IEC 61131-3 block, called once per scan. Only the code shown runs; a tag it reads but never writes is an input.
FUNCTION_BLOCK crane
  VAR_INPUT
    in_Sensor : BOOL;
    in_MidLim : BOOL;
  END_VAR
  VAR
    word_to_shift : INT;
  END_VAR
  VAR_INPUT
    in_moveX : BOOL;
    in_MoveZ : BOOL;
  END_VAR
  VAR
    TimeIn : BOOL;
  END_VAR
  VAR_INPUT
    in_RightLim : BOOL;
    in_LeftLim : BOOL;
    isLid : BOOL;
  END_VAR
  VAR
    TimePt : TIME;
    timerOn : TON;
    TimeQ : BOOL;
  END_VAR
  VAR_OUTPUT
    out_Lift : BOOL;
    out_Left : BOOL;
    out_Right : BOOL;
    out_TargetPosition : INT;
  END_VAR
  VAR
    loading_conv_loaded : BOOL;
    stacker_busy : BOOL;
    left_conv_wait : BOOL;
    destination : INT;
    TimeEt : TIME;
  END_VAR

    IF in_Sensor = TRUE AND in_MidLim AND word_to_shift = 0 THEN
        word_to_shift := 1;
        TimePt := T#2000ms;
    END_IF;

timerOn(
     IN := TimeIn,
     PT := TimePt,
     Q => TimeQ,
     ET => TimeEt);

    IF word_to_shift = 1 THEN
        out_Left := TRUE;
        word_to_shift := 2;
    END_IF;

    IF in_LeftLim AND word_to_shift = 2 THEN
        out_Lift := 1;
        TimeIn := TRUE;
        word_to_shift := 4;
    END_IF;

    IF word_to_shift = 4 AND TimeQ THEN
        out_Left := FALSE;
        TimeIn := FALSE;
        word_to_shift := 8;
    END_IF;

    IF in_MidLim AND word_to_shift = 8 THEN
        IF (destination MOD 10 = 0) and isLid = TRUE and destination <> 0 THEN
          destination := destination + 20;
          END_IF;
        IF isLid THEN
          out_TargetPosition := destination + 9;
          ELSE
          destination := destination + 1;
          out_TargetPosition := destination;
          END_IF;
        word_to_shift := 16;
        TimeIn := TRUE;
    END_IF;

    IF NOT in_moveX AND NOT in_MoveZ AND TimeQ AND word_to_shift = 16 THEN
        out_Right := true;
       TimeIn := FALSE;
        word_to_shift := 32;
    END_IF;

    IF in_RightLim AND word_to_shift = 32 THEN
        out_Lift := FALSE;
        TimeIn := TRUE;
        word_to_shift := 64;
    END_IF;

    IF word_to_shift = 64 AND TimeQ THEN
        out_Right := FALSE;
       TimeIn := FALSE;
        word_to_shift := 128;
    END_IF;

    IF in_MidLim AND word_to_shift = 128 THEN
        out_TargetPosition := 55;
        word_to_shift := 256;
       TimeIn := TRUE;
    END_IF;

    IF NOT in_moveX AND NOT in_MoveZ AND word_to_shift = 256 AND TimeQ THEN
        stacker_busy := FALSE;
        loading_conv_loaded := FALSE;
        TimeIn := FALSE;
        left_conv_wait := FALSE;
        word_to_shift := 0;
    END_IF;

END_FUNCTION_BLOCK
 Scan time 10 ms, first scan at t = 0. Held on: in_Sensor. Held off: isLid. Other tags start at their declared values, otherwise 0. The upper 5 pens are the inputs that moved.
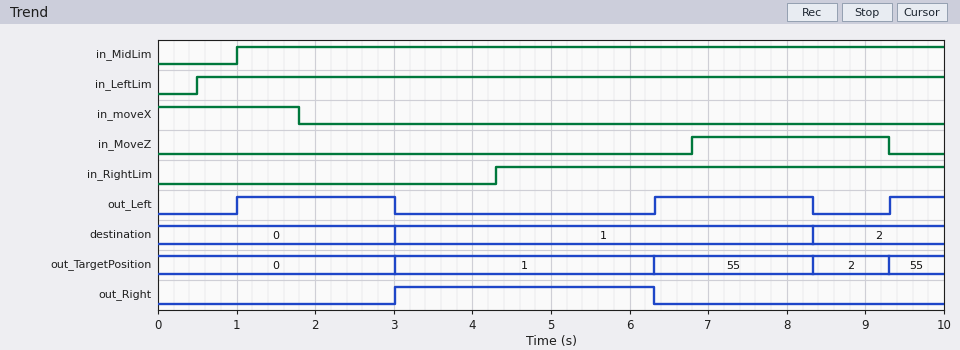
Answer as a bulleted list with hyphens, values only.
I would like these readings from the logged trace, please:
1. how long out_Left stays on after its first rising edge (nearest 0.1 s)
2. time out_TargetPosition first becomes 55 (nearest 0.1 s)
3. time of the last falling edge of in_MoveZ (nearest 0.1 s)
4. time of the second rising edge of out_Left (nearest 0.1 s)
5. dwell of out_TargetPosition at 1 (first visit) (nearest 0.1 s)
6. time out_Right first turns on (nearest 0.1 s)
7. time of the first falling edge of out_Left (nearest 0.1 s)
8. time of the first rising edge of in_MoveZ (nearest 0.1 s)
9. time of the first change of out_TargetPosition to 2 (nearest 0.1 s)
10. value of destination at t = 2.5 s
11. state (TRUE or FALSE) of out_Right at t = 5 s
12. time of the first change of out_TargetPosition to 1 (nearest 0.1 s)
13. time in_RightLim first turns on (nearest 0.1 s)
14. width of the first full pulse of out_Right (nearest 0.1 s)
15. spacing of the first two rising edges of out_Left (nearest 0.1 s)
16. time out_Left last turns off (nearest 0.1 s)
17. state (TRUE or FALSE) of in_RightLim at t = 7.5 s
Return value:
- 2.0 s
- 6.3 s
- 9.3 s
- 6.3 s
- 3.3 s
- 3.0 s
- 3.0 s
- 6.8 s
- 8.3 s
- 0
- TRUE
- 3.0 s
- 4.3 s
- 3.3 s
- 5.3 s
- 8.3 s
- TRUE
